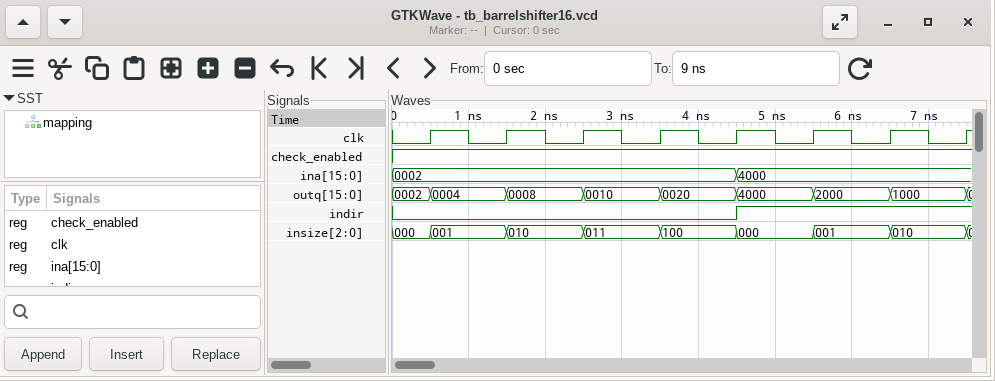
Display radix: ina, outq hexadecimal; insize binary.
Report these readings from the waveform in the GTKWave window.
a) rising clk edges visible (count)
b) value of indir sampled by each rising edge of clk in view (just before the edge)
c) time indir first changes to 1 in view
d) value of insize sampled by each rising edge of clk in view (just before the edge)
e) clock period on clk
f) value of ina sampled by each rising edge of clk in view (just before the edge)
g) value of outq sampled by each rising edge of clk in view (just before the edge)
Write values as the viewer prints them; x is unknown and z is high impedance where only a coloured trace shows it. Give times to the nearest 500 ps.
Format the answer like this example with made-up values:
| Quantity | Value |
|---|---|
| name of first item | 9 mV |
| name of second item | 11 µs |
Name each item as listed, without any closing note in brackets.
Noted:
| Quantity | Value |
|---|---|
| rising clk edges visible | 8 |
| value of indir sampled by each rising edge of clk in view | 0 0 0 0 0 1 1 1 |
| time indir first changes to 1 in view | 4500 ps |
| value of insize sampled by each rising edge of clk in view | 000, 001, 010, 011, 100, 000, 001, 010 |
| clock period on clk | 1000 ps |
| value of ina sampled by each rising edge of clk in view | 0002, 0002, 0002, 0002, 0002, 4000, 4000, 4000 |
| value of outq sampled by each rising edge of clk in view | 0002, 0004, 0008, 0010, 0020, 4000, 2000, 1000 |
